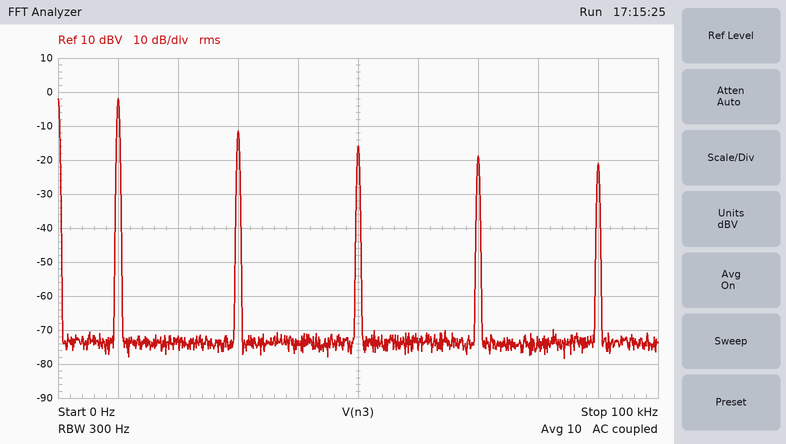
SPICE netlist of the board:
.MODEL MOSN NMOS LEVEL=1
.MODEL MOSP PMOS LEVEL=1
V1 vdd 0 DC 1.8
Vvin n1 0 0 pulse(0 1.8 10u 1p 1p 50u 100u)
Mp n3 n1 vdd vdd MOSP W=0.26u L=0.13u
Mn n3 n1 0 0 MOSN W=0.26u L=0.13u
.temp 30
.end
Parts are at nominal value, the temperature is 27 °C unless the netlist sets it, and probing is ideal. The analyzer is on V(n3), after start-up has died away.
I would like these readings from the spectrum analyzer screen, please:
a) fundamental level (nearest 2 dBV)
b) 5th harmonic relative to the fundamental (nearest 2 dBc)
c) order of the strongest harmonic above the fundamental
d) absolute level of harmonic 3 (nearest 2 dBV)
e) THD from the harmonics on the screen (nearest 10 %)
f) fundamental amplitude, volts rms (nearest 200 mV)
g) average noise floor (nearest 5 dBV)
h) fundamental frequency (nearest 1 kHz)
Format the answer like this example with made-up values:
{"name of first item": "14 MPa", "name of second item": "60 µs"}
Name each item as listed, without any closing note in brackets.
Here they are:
{"fundamental level": "-2 dBV", "5th harmonic relative to the fundamental": "-14 dBc", "order of the strongest harmonic above the fundamental": "3", "absolute level of harmonic 3": "-12 dBV", "THD from the harmonics on the screen": "40 %", "fundamental amplitude, volts rms": "800 mV", "average noise floor": "-75 dBV", "fundamental frequency": "10 kHz"}
